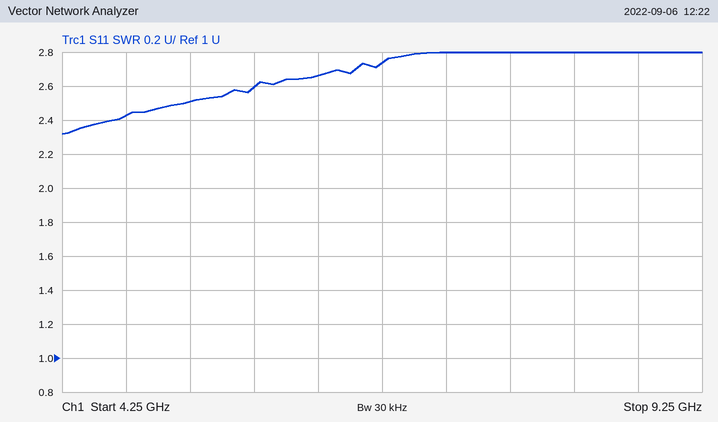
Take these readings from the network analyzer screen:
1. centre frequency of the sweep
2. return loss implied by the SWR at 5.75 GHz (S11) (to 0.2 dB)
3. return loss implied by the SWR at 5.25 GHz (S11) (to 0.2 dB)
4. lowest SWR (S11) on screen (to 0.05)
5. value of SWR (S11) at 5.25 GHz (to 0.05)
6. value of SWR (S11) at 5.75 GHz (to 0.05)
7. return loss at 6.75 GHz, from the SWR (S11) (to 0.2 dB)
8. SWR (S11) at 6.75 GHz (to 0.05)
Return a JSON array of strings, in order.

["6.75 GHz", "7.0 dB", "7.4 dB", "2.30", "2.50", "2.60", "6.6 dB", "2.75"]
